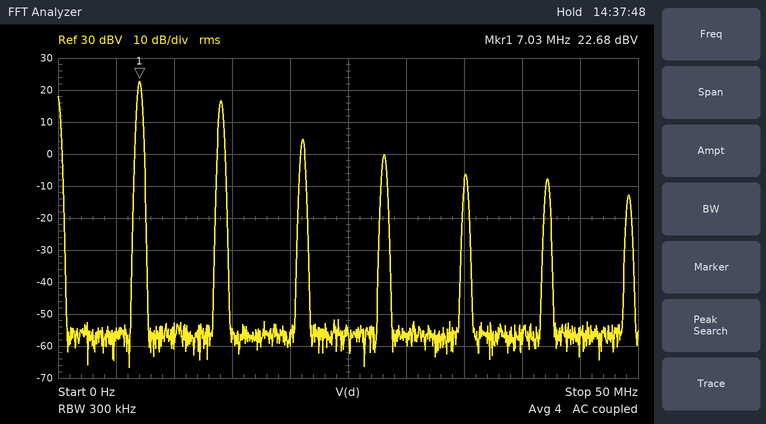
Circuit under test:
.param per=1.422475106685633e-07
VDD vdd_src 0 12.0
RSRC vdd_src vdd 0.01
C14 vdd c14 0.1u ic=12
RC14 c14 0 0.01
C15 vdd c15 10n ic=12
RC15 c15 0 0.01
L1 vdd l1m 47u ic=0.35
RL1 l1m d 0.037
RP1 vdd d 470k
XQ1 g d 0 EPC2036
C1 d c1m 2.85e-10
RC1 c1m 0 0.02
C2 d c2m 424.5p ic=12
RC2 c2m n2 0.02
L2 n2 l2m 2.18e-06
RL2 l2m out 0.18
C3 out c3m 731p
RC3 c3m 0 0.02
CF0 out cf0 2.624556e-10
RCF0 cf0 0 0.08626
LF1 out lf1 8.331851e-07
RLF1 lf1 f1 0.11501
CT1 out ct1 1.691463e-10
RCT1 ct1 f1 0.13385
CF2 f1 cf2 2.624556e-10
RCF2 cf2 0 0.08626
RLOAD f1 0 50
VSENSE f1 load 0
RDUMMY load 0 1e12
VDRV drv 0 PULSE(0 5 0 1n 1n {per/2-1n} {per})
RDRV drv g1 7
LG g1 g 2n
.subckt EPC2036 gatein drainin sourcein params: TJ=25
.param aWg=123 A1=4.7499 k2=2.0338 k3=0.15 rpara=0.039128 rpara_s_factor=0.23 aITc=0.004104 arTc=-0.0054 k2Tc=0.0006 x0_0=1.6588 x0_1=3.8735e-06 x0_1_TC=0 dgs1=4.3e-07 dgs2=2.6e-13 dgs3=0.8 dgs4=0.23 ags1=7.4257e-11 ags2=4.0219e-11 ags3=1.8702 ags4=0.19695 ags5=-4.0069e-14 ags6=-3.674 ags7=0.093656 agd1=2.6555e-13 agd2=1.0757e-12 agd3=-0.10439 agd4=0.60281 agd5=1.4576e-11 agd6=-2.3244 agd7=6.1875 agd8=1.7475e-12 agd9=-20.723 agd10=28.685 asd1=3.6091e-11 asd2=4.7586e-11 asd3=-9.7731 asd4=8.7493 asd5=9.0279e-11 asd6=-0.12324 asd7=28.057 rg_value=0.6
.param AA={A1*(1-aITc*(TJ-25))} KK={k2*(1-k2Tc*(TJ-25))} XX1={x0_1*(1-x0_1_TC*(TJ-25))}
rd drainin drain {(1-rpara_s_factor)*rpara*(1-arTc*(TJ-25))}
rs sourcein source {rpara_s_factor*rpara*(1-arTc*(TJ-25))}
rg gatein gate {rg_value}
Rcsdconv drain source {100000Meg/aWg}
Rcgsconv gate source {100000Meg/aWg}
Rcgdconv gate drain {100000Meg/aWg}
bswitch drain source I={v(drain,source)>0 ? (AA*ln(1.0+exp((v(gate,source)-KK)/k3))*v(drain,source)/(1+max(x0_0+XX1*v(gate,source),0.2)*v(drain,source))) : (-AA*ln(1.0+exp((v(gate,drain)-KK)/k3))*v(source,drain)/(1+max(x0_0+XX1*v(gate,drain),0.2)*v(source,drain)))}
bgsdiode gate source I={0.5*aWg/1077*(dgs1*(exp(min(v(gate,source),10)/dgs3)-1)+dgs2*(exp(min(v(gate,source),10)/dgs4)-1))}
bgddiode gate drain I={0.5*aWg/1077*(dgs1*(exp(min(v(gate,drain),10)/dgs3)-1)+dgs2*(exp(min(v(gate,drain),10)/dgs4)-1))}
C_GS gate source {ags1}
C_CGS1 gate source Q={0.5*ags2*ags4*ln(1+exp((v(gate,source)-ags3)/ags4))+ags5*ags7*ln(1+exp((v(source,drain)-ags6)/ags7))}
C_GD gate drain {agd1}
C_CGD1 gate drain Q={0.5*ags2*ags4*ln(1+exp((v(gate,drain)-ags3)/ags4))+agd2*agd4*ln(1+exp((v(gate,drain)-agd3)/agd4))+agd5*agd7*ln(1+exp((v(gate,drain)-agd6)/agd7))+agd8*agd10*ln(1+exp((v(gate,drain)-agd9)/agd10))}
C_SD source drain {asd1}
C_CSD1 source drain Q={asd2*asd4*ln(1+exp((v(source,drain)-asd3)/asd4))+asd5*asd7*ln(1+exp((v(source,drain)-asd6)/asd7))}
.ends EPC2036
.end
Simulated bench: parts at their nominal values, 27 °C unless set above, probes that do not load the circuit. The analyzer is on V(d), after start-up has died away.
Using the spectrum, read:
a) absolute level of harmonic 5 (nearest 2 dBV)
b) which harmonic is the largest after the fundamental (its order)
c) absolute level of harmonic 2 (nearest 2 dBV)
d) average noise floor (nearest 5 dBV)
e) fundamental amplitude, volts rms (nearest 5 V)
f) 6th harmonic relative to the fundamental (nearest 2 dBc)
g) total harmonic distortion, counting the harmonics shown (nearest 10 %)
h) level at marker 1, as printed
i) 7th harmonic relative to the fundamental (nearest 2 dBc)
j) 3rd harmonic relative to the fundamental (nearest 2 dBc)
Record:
-6 dBV
2
16 dBV
-55 dBV
15 V
-30 dBc
50 %
22.68 dBV
-36 dBc
-18 dBc
